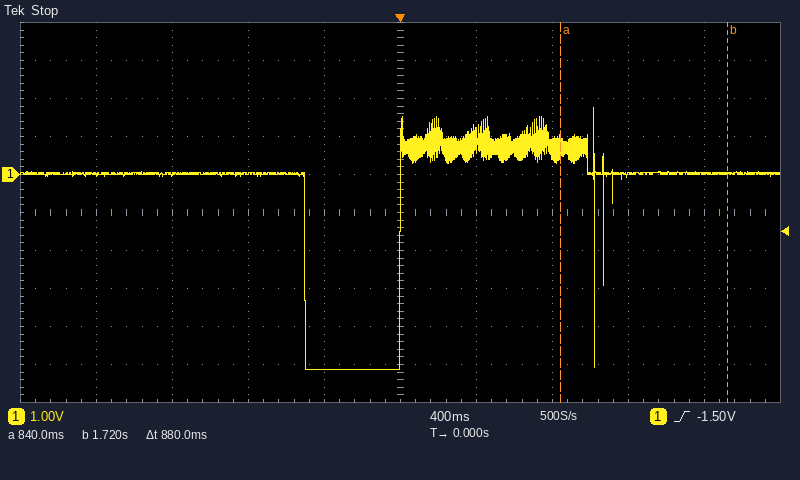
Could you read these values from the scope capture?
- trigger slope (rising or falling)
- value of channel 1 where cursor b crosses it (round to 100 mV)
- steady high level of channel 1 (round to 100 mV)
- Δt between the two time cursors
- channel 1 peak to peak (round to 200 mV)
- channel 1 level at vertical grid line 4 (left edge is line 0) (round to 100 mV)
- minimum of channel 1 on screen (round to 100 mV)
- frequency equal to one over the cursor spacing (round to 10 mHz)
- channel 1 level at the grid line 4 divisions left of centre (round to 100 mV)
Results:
rising
0.0 V
0.0 V
880 ms
6.8 V
-5.1 V
-5.1 V
1.14 Hz
0.0 V
